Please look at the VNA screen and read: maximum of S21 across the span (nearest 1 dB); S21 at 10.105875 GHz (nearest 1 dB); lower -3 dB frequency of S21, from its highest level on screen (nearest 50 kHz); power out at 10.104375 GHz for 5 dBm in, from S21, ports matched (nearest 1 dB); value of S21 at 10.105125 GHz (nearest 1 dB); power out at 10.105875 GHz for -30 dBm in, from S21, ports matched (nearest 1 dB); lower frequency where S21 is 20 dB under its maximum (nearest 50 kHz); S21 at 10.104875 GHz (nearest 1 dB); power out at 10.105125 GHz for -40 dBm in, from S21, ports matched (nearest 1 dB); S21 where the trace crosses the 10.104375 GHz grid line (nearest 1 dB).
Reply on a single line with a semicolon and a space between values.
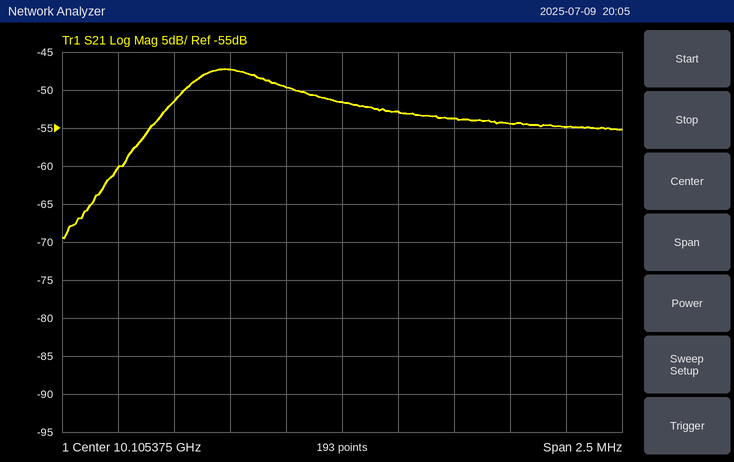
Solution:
-47 dB; -54 dB; 10.10465 GHz; -55 dBm; -50 dB; -84 dBm; 10.10420 GHz; -47 dB; -90 dBm; -60 dB
